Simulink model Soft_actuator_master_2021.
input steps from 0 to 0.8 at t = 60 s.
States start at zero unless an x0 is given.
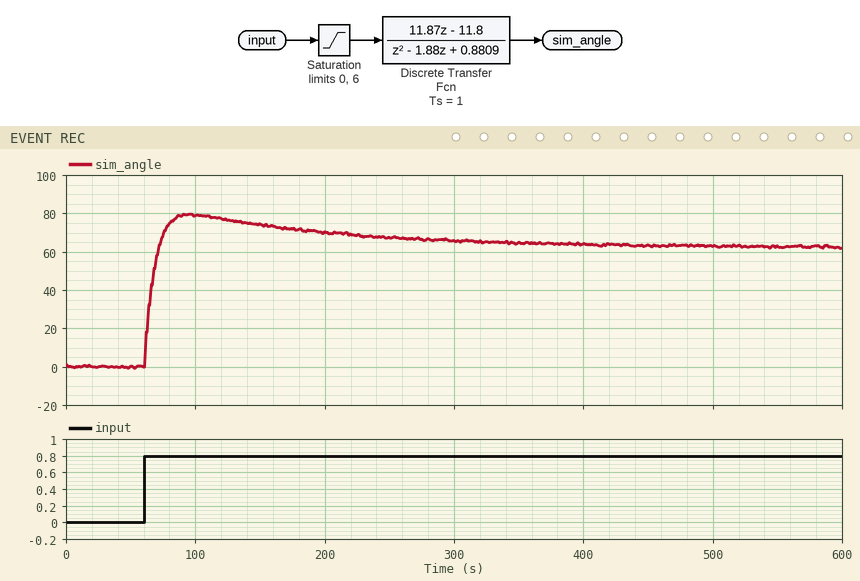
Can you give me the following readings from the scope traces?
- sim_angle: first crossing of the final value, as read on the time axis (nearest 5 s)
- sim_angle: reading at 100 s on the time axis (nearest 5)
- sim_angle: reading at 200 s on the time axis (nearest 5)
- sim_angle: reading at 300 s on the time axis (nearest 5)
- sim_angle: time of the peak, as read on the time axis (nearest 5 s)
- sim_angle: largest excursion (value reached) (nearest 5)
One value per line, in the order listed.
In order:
70 s
80
70
65
95 s
80
